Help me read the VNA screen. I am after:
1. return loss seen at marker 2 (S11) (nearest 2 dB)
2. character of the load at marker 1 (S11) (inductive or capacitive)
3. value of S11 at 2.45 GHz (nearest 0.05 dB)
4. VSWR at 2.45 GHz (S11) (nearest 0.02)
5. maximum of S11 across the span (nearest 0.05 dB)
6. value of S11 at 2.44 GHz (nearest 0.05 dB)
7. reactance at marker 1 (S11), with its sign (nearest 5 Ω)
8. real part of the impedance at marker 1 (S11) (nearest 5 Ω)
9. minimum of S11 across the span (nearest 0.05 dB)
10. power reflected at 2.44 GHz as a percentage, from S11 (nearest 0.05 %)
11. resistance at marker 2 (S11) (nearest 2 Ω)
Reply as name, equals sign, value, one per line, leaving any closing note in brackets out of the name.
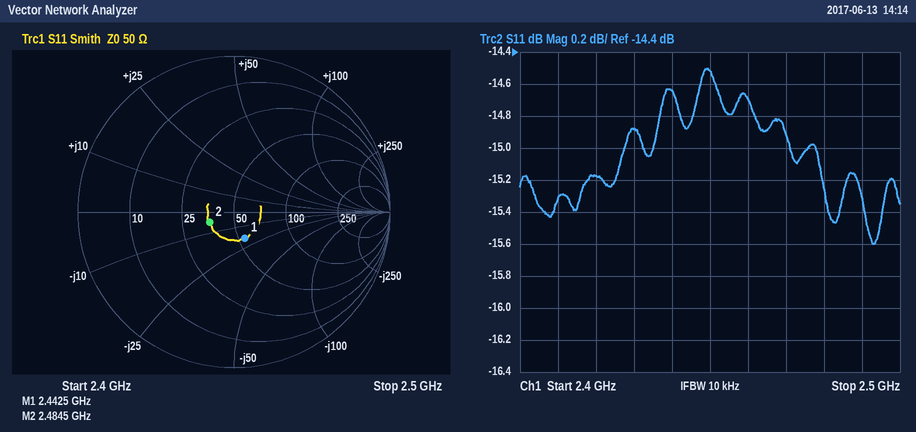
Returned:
return loss seen at marker 2 (S11) = 16 dB
character of the load at marker 1 (S11) = capacitive
value of S11 at 2.45 GHz = -14.50 dB
VSWR at 2.45 GHz (S11) = 1.46
maximum of S11 across the span = -14.50 dB
value of S11 at 2.44 GHz = -14.65 dB
reactance at marker 1 (S11), with its sign = -20 Ω
real part of the impedance at marker 1 (S11) = 55 Ω
minimum of S11 across the span = -15.60 dB
power reflected at 2.44 GHz as a percentage, from S11 = 3.45 %
resistance at marker 2 (S11) = 36 Ω
